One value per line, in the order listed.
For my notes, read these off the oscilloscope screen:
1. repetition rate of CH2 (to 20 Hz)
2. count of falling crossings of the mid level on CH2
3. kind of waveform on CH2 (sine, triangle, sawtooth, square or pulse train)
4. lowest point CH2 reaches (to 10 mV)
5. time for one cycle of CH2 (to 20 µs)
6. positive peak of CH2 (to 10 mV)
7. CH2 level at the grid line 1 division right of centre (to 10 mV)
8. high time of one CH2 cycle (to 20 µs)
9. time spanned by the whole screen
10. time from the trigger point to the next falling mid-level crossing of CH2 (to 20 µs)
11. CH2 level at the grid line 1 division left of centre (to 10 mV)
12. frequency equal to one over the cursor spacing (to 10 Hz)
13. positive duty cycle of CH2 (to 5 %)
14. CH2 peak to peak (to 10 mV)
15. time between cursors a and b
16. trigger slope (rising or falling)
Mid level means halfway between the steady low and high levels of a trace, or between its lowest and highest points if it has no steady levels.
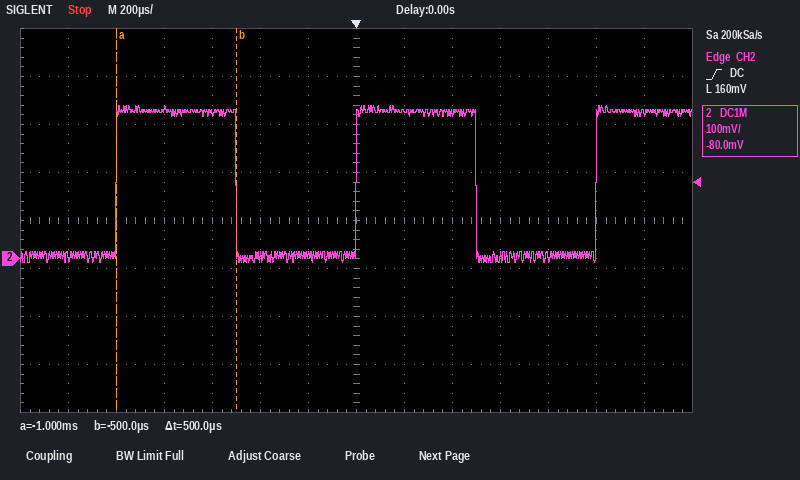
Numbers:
1.00 kHz
2
square
-10 mV
1.00 ms
320 mV
310 mV
500 µs
2.8 ms
500 µs
10 mV
2.00 kHz
50 %
330 mV
500 µs
rising
